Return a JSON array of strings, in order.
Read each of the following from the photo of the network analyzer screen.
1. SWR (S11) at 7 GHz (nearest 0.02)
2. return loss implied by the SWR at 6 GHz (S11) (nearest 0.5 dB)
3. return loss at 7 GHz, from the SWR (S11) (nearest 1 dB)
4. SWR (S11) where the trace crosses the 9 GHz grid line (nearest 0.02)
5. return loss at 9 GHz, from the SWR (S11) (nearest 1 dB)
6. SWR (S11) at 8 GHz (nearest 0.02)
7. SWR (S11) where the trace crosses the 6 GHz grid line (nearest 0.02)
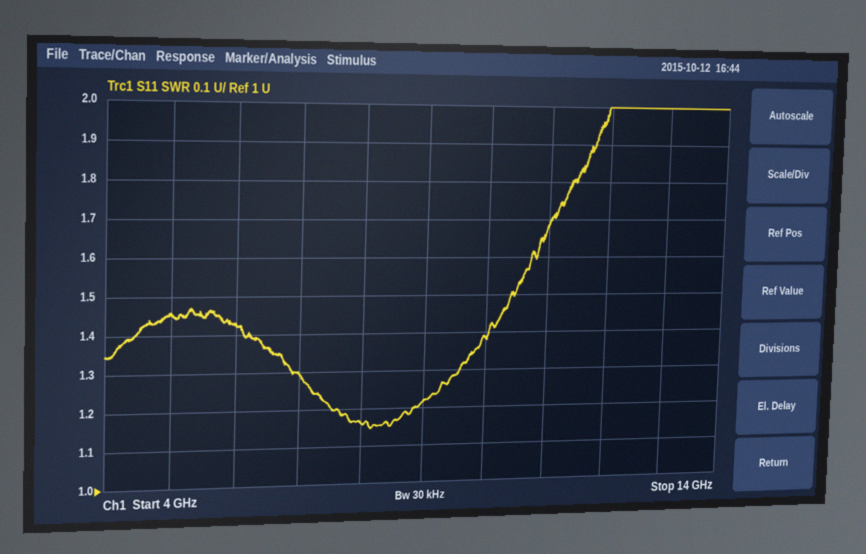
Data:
["1.30", "15.0 dB", "18 dB", "1.22", "20 dB", "1.16", "1.42"]
